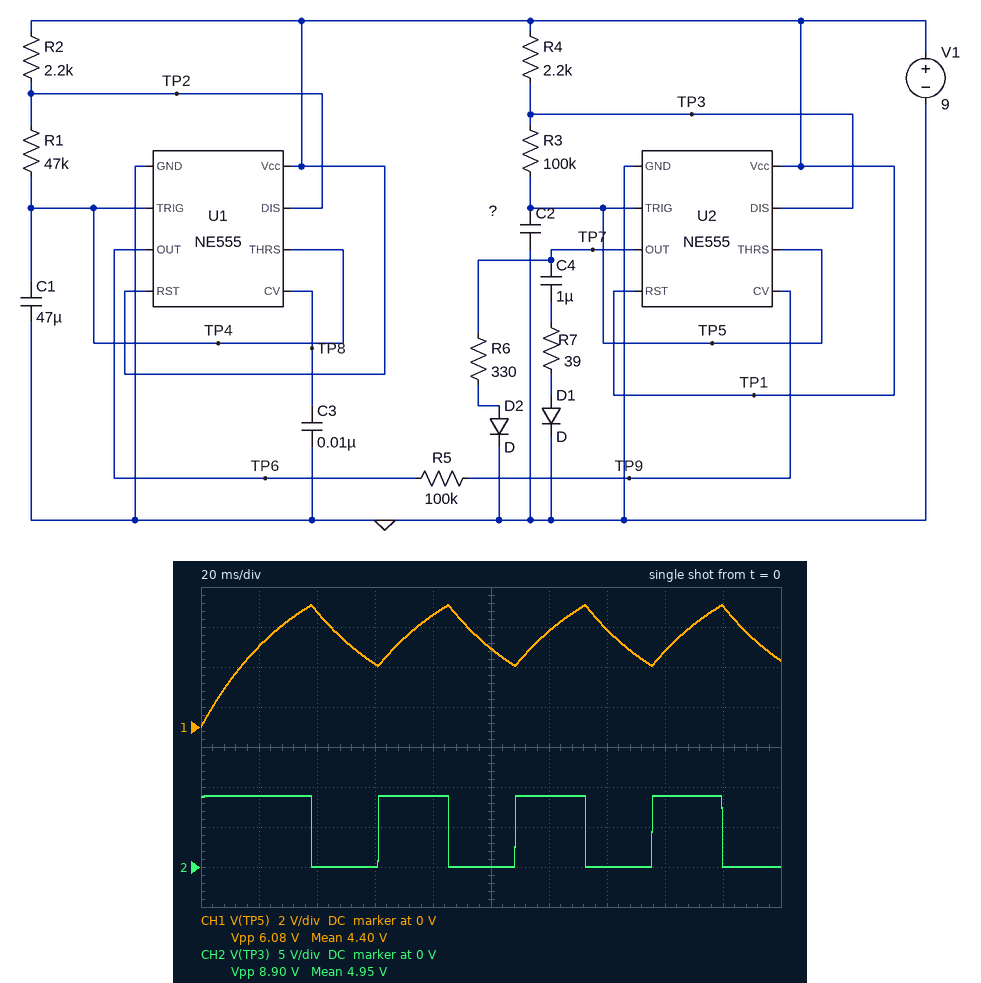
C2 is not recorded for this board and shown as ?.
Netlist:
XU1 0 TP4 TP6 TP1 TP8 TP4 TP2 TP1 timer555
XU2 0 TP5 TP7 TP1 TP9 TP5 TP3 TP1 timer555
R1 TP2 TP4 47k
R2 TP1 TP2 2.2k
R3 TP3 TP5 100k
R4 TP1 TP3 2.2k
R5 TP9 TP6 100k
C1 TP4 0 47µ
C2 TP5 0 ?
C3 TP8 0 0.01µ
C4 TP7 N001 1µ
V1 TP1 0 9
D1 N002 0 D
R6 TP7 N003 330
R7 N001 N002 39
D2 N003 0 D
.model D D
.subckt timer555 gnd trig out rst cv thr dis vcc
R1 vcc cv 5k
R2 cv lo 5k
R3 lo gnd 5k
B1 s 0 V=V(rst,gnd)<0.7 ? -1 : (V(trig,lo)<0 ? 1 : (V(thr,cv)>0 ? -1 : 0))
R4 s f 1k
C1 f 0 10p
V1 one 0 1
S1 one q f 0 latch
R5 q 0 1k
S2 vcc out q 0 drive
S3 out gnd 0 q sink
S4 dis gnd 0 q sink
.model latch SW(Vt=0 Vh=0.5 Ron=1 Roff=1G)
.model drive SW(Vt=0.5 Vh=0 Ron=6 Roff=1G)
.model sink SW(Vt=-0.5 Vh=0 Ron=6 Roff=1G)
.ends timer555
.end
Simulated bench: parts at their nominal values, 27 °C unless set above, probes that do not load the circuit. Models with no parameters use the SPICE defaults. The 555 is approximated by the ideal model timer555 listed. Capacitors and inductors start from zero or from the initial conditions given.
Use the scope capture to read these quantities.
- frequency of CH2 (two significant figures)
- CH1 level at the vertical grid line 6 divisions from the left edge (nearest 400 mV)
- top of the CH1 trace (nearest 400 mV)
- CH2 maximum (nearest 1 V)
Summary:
21 Hz
4.8 V
6.0 V
9 V
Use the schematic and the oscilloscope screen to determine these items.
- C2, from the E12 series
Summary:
330 nF
